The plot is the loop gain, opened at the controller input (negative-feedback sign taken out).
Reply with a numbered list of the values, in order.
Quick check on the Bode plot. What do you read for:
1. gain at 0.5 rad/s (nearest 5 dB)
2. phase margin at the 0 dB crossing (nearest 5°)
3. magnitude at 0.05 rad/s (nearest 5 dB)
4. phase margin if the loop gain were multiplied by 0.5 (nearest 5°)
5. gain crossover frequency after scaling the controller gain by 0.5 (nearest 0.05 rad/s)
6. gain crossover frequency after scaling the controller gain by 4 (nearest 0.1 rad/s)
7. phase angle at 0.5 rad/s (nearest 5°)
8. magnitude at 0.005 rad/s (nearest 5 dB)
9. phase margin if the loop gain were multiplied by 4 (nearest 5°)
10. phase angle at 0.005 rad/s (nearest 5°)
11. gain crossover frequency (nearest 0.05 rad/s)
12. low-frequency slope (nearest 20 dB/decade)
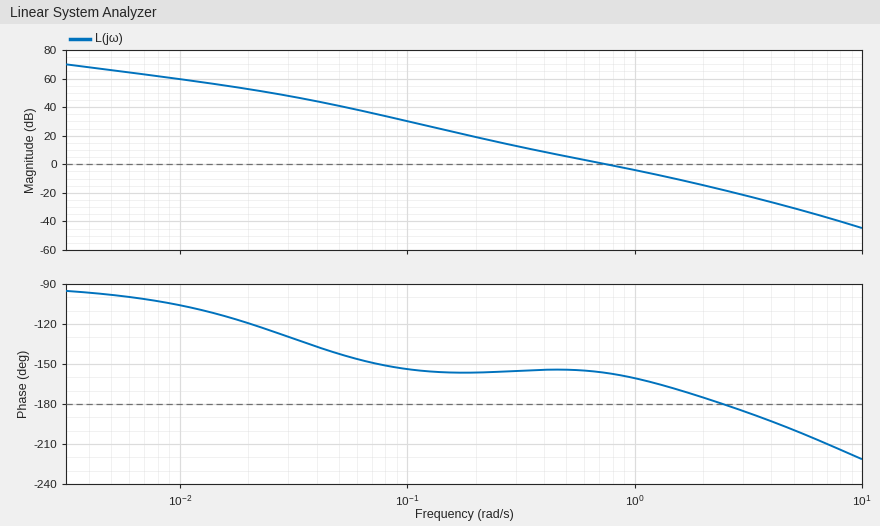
1. 5 dB
2. 25°
3. 40 dB
4. 25°
5. 0.50 rad/s
6. 1.7 rad/s
7. -155°
8. 65 dB
9. 10°
10. -100°
11. 0.75 rad/s
12. -20 dB/decade
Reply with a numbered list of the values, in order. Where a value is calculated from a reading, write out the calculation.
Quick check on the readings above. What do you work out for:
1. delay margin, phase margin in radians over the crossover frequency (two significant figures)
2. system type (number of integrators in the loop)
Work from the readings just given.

1. 25 × π / 180 / 0.75 = 0.58 s
2. 1
